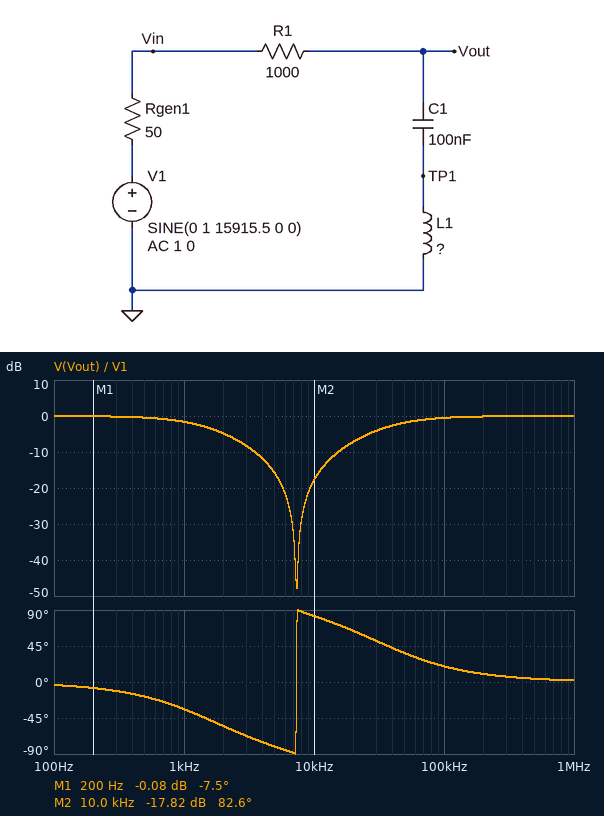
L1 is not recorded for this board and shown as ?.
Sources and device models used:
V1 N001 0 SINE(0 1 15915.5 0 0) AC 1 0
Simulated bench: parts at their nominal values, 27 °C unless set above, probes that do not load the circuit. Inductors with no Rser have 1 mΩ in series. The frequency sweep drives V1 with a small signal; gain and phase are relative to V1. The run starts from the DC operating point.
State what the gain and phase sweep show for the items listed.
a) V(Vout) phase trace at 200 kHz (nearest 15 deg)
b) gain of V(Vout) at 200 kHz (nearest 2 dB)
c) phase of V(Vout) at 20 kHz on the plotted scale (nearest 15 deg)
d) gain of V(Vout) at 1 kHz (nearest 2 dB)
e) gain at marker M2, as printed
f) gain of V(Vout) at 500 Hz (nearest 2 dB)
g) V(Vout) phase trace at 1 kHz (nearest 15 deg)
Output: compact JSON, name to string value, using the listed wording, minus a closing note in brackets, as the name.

{"V(Vout) phase trace at 200 kHz": "15 deg", "gain of V(Vout) at 200 kHz": "0 dB", "phase of V(Vout) at 20 kHz on the plotted scale": "60 deg", "gain of V(Vout) at 1 kHz": "-2 dB", "gain at marker M2, as printed": "-17.82 dB", "gain of V(Vout) at 500 Hz": "0 dB", "V(Vout) phase trace at 1 kHz": "-30 deg"}
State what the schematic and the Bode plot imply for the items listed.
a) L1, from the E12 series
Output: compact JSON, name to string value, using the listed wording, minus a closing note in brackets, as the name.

{"L1, from the E12 series": "4.7 mH"}
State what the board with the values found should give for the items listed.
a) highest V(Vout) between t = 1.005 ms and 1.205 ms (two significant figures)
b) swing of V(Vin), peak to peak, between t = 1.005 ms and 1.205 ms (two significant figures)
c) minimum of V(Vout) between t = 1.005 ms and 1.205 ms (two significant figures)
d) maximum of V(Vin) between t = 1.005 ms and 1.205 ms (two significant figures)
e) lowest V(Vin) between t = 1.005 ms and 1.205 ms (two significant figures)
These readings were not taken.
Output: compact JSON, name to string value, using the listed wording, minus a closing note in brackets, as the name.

{"highest V(Vout) between t = 1.005 ms and 1.205 ms": "330 mV", "swing of V(Vin), peak to peak, between t = 1.005 ms and 1.205 ms": "1.9 V", "minimum of V(Vout) between t = 1.005 ms and 1.205 ms": "-330 mV", "maximum of V(Vin) between t = 1.005 ms and 1.205 ms": "960 mV", "lowest V(Vin) between t = 1.005 ms and 1.205 ms": "-960 mV"}
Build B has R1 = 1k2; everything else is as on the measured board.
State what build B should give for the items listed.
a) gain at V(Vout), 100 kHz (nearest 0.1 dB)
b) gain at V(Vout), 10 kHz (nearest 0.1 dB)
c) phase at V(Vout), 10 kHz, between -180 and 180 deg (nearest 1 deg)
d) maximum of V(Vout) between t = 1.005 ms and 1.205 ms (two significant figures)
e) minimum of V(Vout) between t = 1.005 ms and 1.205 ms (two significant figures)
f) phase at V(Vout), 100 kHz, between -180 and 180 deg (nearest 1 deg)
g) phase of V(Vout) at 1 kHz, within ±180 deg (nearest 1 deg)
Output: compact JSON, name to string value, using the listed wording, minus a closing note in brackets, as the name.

{"gain at V(Vout), 100 kHz": "-0.7 dB", "gain at V(Vout), 10 kHz": "-19.3 dB", "phase at V(Vout), 10 kHz, between -180 and 180 deg": "84 deg", "maximum of V(Vout) between t = 1.005 ms and 1.205 ms": "280 mV", "minimum of V(Vout) between t = 1.005 ms and 1.205 ms": "-280 mV", "phase at V(Vout), 100 kHz, between -180 and 180 deg": "23 deg", "phase of V(Vout) at 1 kHz, within ±180 deg": "-39 deg"}
